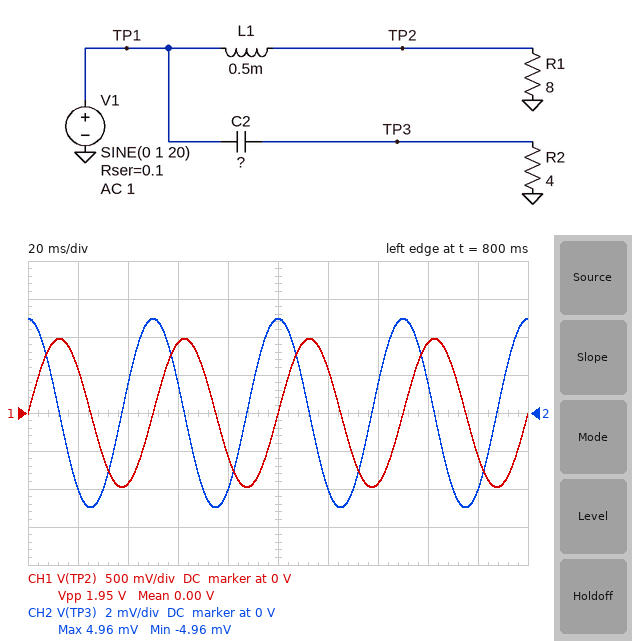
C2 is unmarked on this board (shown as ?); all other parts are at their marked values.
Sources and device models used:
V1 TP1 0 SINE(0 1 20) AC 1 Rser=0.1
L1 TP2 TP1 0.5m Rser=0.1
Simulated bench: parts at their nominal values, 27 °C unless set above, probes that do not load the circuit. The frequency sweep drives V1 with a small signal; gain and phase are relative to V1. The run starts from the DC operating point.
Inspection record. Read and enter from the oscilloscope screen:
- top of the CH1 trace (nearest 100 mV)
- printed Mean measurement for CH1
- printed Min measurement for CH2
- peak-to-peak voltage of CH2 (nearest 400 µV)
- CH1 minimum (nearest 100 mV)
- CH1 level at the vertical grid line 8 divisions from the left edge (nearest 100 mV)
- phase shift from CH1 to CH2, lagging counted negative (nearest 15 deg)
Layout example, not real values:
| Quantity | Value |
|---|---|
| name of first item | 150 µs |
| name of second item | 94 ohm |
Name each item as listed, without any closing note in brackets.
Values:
| Quantity | Value |
|---|---|
| top of the CH1 trace | 1.0 V |
| printed Mean measurement for CH1 | 0.00 V |
| printed Min measurement for CH2 | -4.96 mV |
| peak-to-peak voltage of CH2 | 10.0 mV |
| CH1 minimum | -1.0 V |
| CH1 level at the vertical grid line 8 divisions from the left edge | 900 mV |
| phase shift from CH1 to CH2, lagging counted negative | 90 deg |
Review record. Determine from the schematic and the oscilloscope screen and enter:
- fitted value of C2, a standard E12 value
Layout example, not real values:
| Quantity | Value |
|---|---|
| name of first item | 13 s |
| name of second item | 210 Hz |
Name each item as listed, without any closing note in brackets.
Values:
| Quantity | Value |
|---|---|
| fitted value of C2, a standard E12 value | 10 µF |
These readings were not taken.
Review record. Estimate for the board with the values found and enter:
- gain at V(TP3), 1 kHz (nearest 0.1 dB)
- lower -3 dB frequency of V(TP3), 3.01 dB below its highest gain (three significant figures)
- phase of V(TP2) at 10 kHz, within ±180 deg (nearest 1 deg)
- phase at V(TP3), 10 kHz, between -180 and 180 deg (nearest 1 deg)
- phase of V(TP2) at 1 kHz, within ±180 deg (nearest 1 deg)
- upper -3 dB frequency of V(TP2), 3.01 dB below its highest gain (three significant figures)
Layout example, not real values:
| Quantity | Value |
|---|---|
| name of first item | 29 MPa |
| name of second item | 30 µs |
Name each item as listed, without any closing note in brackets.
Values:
| Quantity | Value |
|---|---|
| gain at V(TP3), 1 kHz | -12.4 dB |
| lower -3 dB frequency of V(TP3), 3.01 dB below its highest gain | 3.91 kHz |
| phase of V(TP2) at 10 kHz, within ±180 deg | -76 deg |
| phase at V(TP3), 10 kHz, between -180 and 180 deg | 21 deg |
| phase of V(TP2) at 1 kHz, within ±180 deg | -21 deg |
| upper -3 dB frequency of V(TP2), 3.01 dB below its highest gain | 2.57 kHz |
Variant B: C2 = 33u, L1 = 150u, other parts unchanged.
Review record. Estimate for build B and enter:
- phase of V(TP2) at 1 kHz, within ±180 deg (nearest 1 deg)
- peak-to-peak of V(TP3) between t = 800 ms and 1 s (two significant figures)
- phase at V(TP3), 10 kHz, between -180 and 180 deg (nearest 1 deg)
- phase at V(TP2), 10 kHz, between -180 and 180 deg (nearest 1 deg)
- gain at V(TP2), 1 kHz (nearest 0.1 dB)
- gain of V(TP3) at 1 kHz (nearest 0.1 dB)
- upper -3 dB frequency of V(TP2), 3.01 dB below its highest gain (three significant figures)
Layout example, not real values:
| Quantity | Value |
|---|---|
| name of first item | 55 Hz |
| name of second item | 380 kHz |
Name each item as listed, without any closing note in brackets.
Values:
| Quantity | Value |
|---|---|
| phase of V(TP2) at 1 kHz, within ±180 deg | -7 deg |
| peak-to-peak of V(TP3) between t = 800 ms and 1 s | 33 mV |
| phase at V(TP3), 10 kHz, between -180 and 180 deg | 7 deg |
| phase at V(TP2), 10 kHz, between -180 and 180 deg | -49 deg |
| gain at V(TP2), 1 kHz | -0.4 dB |
| gain of V(TP3) at 1 kHz | -4.1 dB |
| upper -3 dB frequency of V(TP2), 3.01 dB below its highest gain | 8.28 kHz |
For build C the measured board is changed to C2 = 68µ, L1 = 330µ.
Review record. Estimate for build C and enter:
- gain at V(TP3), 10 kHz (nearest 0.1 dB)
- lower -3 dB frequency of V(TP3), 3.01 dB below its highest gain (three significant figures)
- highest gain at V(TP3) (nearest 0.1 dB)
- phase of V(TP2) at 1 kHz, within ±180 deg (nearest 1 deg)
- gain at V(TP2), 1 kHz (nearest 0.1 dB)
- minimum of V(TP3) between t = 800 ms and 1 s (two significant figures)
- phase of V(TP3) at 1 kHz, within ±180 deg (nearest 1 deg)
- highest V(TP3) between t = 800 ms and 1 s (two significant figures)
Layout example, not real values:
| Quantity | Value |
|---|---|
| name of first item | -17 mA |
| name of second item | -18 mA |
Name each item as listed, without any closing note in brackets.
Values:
| Quantity | Value |
|---|---|
| gain at V(TP3), 10 kHz | -0.2 dB |
| lower -3 dB frequency of V(TP3), 3.01 dB below its highest gain | 585 Hz |
| highest gain at V(TP3) | -0.2 dB |
| phase of V(TP2) at 1 kHz, within ±180 deg | -15 deg |
| gain at V(TP2), 1 kHz | -0.6 dB |
| minimum of V(TP3) between t = 800 ms and 1 s | -34 mV |
| phase of V(TP3) at 1 kHz, within ±180 deg | 30 deg |
| highest V(TP3) between t = 800 ms and 1 s | 34 mV |
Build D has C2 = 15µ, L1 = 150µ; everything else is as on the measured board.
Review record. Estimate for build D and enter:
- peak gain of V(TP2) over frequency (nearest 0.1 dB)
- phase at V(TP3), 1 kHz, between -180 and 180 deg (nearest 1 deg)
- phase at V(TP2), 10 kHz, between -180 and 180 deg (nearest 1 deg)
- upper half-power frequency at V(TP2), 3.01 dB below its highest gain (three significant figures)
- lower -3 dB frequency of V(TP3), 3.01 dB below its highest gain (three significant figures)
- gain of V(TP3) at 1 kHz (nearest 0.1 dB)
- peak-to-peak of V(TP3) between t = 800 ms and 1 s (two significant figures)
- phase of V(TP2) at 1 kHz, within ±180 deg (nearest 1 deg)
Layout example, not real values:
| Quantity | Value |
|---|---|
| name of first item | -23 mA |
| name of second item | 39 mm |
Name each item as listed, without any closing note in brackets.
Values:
| Quantity | Value |
|---|---|
| peak gain of V(TP2) over frequency | -0.2 dB |
| phase at V(TP3), 1 kHz, between -180 and 180 deg | 69 deg |
| phase at V(TP2), 10 kHz, between -180 and 180 deg | -49 deg |
| upper half-power frequency at V(TP2), 3.01 dB below its highest gain | 8.31 kHz |
| lower -3 dB frequency of V(TP3), 3.01 dB below its highest gain | 2.65 kHz |
| gain of V(TP3) at 1 kHz | -9.2 dB |
| peak-to-peak of V(TP3) between t = 800 ms and 1 s | 15 mV |
| phase of V(TP2) at 1 kHz, within ±180 deg | -7 deg |
